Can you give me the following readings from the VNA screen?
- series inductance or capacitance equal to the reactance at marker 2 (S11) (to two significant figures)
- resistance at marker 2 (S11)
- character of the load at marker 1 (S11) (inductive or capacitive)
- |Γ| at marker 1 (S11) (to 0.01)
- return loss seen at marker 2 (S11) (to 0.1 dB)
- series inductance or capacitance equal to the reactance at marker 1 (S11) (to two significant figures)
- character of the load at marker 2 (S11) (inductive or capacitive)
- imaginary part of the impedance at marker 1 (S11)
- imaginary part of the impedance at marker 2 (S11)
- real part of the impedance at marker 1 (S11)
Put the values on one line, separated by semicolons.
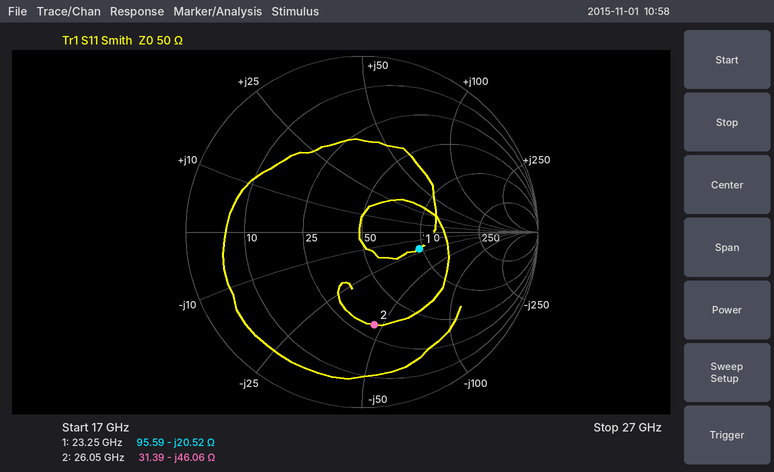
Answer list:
130 fF; 31.39 Ω; capacitive; 0.34; 5.5 dB; 330 fF; capacitive; -20.52 Ω; -46.06 Ω; 95.59 Ω
